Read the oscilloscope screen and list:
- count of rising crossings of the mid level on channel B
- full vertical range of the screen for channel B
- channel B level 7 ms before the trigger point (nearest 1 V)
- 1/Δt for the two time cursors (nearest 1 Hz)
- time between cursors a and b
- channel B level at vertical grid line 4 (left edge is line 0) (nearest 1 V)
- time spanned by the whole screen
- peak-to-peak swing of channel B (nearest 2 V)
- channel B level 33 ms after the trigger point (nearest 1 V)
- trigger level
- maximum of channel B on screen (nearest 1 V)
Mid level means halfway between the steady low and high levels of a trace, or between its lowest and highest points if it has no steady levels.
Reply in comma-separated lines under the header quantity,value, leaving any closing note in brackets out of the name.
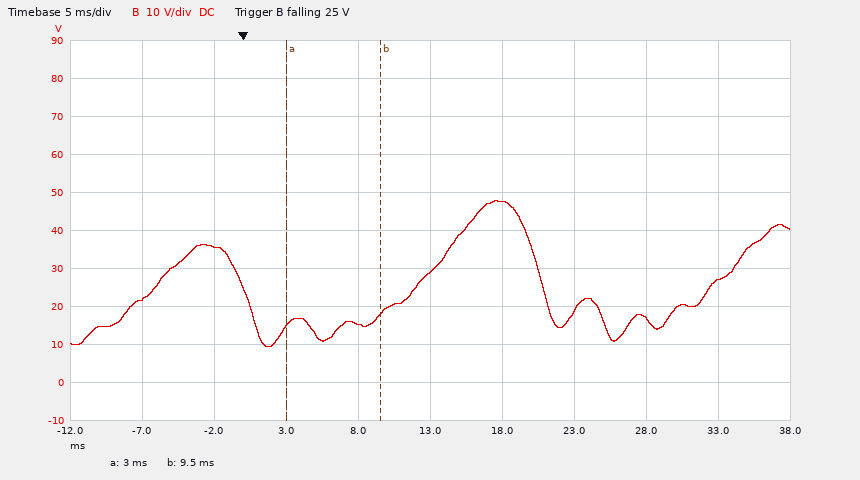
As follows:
quantity,value
count of rising crossings of the mid level on channel B,3
full vertical range of the screen for channel B,100 V
channel B level 7 ms before the trigger point,22 V
1/Δt for the two time cursors,154 Hz
time between cursors a and b,6.5 ms
channel B level at vertical grid line 4 (left edge is line 0),15 V
time spanned by the whole screen,50 ms
peak-to-peak swing of channel B,38 V
channel B level 33 ms after the trigger point,27 V
trigger level,25 V
maximum of channel B on screen,48 V
